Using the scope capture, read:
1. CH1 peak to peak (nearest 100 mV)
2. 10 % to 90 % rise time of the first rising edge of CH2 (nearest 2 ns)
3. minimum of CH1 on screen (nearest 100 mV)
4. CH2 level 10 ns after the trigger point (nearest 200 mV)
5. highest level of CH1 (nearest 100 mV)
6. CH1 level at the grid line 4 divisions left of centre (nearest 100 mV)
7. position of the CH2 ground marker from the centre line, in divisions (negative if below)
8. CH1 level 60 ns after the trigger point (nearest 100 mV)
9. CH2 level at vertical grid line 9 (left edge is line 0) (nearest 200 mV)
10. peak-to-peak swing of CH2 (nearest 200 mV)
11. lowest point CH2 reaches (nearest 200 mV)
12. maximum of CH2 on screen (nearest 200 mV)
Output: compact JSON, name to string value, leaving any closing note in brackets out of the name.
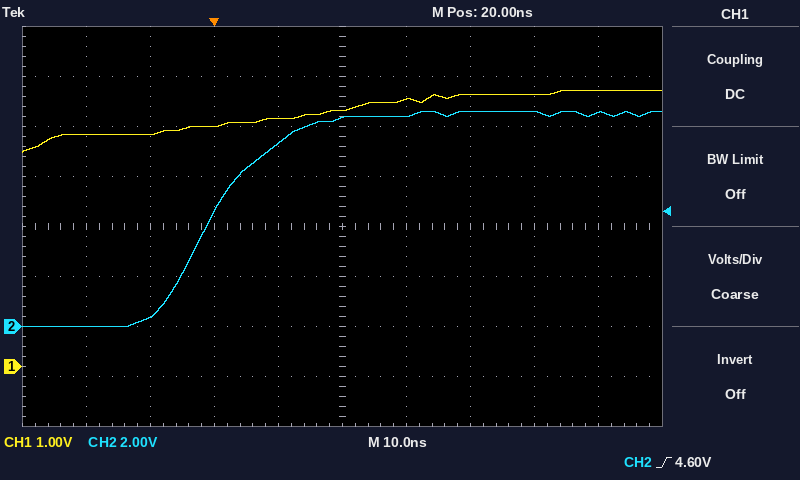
{"CH1 peak to peak": "1.2 V", "10 % to 90 % rise time of the first rising edge of CH2": "20 ns", "minimum of CH1 on screen": "4.3 V", "CH2 level 10 ns after the trigger point": "7.4 V", "highest level of CH1": "5.5 V", "CH1 level at the grid line 4 divisions left of centre": "4.6 V", "position of the CH2 ground marker from the centre line, in divisions": "-2.0 div", "CH1 level 60 ns after the trigger point": "5.5 V", "CH2 level at vertical grid line 9 (left edge is line 0)": "8.6 V", "peak-to-peak swing of CH2": "8.6 V", "lowest point CH2 reaches": "0.0 V", "maximum of CH2 on screen": "8.6 V"}
